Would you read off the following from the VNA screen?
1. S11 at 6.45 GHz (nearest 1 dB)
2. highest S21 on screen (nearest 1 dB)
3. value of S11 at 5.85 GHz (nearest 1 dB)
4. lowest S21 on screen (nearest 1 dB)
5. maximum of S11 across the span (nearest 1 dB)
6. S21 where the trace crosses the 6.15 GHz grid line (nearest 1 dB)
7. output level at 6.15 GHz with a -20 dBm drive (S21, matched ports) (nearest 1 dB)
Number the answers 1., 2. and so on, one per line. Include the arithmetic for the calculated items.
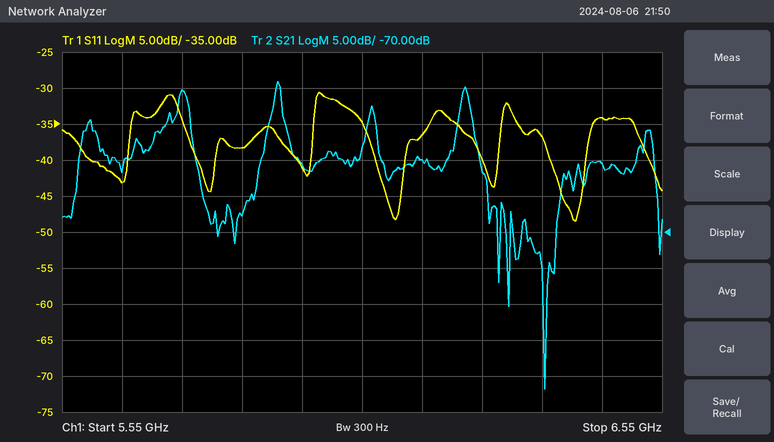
1. -34 dB
2. -49 dB
3. -38 dB
4. -92 dB
5. -31 dB
6. -60 dB
7. -20 dBm + (-60 dB) = -80 dBm
